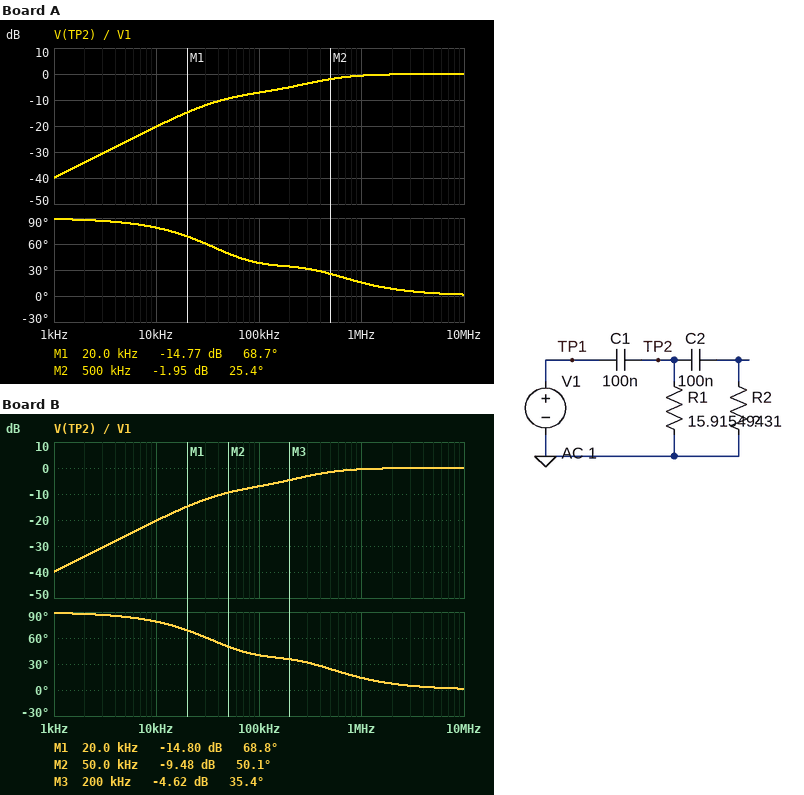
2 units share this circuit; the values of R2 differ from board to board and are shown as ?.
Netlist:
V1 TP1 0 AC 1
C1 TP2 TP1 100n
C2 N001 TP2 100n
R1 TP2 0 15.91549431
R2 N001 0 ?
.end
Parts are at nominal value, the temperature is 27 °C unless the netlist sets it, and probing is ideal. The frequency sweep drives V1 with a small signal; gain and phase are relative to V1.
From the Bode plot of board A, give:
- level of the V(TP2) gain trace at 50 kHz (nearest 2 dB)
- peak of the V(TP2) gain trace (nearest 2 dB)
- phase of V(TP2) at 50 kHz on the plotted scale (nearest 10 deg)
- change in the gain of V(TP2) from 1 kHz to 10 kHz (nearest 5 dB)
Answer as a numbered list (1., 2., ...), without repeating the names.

1. -10 dB
2. 0 dB
3. 50 deg
4. 20 dB
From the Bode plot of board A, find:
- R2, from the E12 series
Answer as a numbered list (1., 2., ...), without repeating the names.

1. 8.2 Ω
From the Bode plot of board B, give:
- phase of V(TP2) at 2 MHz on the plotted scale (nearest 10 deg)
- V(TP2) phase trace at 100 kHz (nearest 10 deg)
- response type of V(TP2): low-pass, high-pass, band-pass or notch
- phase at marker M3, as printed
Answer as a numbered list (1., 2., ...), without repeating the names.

1. 10 deg
2. 40 deg
3. high-pass
4. 35.4 deg
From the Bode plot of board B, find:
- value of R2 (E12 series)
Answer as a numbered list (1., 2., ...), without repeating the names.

1. 10 Ω
